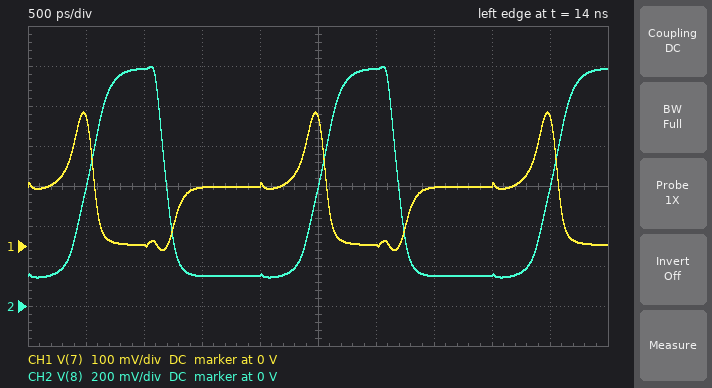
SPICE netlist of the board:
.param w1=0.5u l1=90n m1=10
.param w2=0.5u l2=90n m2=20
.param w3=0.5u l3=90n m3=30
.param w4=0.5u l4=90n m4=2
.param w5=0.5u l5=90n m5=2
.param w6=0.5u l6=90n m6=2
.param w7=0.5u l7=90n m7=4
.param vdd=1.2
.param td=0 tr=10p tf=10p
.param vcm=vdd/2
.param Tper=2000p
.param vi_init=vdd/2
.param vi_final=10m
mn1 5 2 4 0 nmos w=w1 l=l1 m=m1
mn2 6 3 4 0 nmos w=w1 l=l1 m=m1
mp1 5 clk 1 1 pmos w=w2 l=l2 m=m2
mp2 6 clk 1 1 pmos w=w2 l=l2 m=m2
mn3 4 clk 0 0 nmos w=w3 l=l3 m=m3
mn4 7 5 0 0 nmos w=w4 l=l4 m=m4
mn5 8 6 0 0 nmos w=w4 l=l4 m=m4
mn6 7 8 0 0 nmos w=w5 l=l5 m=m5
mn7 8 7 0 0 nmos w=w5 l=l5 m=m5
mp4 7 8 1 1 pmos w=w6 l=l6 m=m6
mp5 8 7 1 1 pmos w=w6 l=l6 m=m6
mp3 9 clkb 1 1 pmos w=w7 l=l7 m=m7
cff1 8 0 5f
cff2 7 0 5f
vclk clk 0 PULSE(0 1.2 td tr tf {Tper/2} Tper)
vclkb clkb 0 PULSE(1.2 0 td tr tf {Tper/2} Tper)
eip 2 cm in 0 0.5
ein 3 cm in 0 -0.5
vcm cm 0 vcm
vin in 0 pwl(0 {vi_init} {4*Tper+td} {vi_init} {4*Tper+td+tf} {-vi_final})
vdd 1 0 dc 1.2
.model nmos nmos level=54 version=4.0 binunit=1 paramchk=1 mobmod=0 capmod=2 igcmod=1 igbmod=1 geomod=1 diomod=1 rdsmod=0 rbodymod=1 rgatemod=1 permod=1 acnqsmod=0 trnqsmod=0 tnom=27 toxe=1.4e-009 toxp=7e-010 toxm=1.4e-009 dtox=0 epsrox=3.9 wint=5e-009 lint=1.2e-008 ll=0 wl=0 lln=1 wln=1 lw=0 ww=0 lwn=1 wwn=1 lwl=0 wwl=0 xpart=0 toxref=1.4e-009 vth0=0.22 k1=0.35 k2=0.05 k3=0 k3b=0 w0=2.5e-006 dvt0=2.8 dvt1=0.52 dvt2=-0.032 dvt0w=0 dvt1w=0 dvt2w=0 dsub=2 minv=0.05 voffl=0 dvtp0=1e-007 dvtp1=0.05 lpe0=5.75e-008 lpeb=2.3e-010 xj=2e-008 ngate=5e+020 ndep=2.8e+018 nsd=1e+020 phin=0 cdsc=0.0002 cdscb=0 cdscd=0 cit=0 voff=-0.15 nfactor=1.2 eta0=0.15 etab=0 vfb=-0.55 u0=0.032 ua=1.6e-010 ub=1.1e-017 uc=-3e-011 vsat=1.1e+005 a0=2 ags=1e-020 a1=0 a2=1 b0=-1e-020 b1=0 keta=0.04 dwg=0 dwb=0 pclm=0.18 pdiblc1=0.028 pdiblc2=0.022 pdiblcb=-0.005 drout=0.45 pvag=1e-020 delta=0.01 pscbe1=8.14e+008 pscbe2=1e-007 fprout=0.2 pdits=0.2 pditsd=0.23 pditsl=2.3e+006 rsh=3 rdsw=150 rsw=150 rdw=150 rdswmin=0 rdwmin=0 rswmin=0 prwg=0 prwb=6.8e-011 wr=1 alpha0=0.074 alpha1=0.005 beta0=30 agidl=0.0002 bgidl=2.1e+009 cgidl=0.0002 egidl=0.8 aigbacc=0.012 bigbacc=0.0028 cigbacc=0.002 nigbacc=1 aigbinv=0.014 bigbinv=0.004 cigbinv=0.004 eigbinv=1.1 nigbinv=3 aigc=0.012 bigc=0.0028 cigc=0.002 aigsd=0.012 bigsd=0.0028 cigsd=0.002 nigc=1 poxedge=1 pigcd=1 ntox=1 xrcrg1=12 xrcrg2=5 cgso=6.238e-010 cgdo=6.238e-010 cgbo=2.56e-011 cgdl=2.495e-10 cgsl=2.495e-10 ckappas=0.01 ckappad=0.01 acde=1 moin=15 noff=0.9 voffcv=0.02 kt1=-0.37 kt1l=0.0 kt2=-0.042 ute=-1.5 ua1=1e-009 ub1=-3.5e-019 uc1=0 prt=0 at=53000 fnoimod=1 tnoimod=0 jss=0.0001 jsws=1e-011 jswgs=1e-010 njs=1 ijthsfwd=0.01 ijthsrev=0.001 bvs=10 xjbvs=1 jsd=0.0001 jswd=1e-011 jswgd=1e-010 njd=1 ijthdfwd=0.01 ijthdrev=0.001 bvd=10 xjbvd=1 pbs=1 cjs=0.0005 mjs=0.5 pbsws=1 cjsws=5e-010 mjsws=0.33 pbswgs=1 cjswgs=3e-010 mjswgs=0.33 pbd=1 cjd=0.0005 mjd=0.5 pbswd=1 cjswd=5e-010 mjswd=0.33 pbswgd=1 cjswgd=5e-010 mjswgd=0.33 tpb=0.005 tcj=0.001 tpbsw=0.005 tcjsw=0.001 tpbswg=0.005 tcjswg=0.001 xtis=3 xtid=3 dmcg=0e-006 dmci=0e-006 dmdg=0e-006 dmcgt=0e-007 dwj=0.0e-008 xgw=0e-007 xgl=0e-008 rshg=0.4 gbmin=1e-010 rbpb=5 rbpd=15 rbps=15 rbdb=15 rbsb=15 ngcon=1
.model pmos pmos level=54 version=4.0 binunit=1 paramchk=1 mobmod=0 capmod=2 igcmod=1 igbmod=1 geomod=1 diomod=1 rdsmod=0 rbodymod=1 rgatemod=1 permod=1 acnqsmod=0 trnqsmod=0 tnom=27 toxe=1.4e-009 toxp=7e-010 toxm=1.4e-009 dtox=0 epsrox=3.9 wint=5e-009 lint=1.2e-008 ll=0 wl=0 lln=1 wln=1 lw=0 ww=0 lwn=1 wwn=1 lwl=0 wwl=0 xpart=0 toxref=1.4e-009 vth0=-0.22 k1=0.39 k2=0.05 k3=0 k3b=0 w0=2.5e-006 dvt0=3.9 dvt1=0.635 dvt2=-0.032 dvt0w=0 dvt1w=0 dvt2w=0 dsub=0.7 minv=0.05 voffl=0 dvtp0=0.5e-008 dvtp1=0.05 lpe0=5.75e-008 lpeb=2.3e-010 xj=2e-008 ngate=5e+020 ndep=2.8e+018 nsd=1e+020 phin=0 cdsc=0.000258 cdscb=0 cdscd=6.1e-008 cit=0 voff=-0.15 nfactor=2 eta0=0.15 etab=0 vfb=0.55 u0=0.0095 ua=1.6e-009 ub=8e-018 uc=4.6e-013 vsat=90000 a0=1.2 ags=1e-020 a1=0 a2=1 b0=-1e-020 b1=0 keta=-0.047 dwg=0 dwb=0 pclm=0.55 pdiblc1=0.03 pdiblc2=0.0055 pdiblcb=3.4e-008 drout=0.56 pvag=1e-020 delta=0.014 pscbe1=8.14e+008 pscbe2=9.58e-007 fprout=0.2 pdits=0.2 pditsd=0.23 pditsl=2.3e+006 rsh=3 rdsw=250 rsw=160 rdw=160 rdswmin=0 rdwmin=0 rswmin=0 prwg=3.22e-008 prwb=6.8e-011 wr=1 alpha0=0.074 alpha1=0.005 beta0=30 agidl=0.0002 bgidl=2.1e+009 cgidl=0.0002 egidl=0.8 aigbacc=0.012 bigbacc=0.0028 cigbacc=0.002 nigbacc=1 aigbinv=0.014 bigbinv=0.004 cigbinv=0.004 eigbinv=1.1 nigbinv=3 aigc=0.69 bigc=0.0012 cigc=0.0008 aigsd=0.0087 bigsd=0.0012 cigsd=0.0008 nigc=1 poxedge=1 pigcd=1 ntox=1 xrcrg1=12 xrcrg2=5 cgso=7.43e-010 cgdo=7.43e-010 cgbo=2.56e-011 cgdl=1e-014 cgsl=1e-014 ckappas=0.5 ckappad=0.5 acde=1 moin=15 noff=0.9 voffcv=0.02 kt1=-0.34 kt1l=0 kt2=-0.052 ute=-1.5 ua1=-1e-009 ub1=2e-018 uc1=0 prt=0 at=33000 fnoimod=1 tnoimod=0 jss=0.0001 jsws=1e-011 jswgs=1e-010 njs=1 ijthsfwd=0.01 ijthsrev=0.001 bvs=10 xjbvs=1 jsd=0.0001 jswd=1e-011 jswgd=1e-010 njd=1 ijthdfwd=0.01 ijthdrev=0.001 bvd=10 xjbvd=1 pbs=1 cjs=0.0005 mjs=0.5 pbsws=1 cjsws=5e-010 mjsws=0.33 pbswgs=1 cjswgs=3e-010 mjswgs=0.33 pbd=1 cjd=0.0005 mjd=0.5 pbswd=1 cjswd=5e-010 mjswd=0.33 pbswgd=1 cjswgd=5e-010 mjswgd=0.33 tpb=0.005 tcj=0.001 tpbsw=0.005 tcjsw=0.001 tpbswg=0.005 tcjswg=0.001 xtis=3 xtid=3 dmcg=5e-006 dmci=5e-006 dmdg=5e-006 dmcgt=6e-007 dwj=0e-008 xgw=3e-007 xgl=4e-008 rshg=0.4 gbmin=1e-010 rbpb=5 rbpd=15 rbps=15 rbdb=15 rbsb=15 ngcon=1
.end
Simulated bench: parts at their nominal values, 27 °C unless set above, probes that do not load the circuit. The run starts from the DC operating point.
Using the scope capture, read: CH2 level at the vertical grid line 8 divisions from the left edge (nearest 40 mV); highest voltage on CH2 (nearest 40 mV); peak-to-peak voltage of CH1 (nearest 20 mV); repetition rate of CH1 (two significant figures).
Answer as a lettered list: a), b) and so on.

a) 160 mV
b) 1.20 V
c) 340 mV
d) 500 MHz
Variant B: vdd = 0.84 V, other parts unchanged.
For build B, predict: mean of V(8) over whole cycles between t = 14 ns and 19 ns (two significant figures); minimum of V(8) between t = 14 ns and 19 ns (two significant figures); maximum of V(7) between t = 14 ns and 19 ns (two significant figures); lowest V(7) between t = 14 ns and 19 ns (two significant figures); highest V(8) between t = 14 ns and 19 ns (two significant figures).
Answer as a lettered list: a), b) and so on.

a) 360 mV
b) 77 mV
c) 280 mV
d) -9.4 mV
e) 840 mV
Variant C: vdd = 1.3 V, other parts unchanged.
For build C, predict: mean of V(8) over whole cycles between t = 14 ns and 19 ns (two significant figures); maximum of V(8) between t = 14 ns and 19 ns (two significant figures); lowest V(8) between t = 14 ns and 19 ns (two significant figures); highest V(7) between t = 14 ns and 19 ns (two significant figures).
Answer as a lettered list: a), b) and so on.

a) 520 mV
b) 1.3 V
c) 160 mV
d) 340 mV
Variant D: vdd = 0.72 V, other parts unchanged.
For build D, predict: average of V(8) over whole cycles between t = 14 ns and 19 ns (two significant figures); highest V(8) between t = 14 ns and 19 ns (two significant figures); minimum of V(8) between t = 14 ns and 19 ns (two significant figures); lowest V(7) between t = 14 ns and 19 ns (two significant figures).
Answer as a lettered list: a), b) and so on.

a) 280 mV
b) 670 mV
c) 57 mV
d) -7.9 mV
